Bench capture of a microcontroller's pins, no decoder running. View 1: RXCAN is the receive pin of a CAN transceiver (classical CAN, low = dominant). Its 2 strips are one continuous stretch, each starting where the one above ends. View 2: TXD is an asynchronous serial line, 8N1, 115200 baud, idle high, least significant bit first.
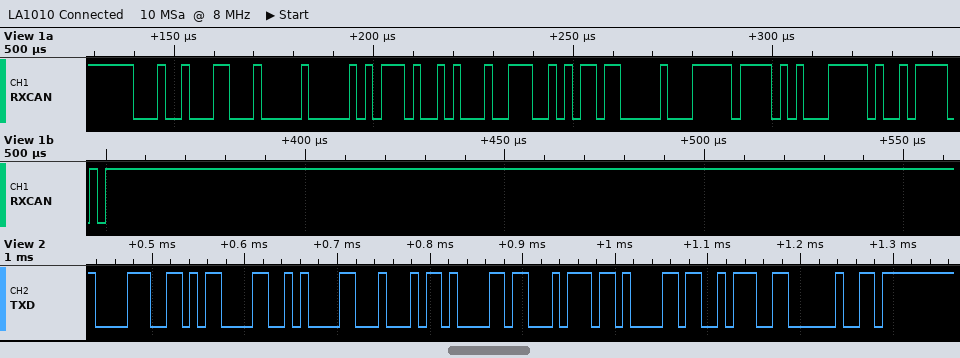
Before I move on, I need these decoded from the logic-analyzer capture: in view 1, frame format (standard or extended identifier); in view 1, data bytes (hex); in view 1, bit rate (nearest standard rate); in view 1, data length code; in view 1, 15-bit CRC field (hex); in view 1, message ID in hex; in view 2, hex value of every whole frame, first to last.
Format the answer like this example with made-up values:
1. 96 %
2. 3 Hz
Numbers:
1. standard
2. 00 BA 51 39 5B 00 FF A8
3. 500 kbit/s
4. 8
5. 0x7E5E
6. 0x123
7. 38 0D 0A 44 61 74 61 3A 20 FF
